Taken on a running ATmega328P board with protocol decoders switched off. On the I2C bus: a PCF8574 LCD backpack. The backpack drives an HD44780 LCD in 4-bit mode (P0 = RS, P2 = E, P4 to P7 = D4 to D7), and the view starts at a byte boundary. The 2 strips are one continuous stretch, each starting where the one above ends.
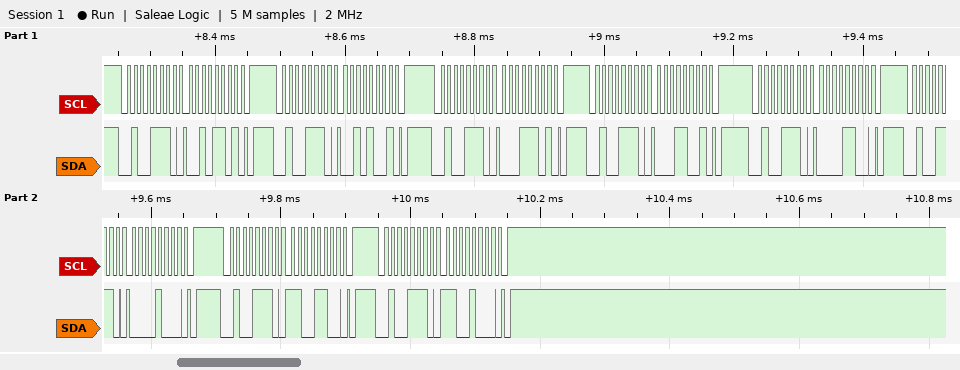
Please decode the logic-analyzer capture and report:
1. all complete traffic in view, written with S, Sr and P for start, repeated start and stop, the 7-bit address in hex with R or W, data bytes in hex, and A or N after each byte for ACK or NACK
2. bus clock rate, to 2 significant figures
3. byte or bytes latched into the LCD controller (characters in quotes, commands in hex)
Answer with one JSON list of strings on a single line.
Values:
["S 27W A 2D A P S 27W A 29 A P S 27W A 1D A P S 27W A 19 A P S 27W A 0C A P S 27W A 08 A P S 27W A CC A P S 27W A C8 A P", "100 kHz", "'!' 0x0C"]
